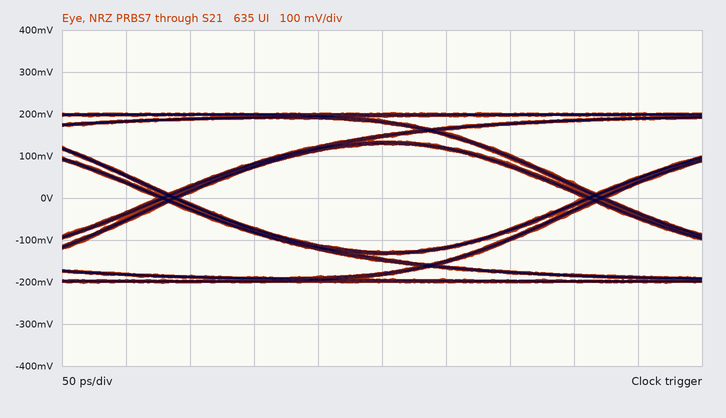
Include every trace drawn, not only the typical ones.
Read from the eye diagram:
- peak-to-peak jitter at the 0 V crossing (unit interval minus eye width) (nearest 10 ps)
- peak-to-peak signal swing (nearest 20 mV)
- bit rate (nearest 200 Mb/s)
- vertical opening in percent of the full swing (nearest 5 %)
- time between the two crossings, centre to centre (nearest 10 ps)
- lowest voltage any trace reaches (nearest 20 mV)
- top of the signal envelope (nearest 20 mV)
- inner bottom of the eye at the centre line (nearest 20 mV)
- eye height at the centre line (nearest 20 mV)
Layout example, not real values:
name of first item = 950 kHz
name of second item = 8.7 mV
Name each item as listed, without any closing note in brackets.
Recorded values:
peak-to-peak jitter at the 0 V crossing (unit interval minus eye width) = 20 ps
peak-to-peak signal swing = 400 mV
bit rate = 3.0 Gb/s
vertical opening in percent of the full swing = 65 %
time between the two crossings, centre to centre = 330 ps
lowest voltage any trace reaches = -200 mV
top of the signal envelope = 200 mV
inner bottom of the eye at the centre line = -120 mV
eye height at the centre line = 260 mV
